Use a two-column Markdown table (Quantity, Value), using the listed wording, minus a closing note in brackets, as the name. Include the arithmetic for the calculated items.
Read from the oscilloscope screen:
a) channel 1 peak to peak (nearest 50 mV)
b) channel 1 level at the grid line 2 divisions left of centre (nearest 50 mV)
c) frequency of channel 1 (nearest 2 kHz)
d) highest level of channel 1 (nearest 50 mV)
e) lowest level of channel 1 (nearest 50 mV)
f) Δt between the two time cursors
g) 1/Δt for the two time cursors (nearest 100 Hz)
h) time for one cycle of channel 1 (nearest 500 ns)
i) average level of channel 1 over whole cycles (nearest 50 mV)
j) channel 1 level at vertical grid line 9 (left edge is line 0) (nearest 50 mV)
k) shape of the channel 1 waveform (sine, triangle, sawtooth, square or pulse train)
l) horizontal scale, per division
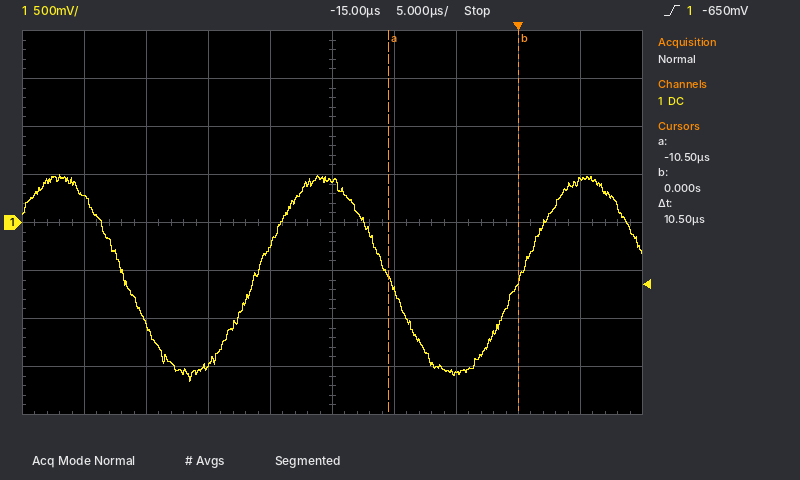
| Quantity | Value |
|---|---|
| channel 1 peak to peak | 500 mV − (-1.65 V) = 2.15 V |
| channel 1 level at the grid line 2 divisions left of centre | -1.50 V |
| frequency of channel 1 | 1 / 21.5 µs ≈ 46 kHz |
| highest level of channel 1 | 500 mV |
| lowest level of channel 1 | -1.65 V |
| Δt between the two time cursors | 10.5 µs |
| 1/Δt for the two time cursors | 1 / 10.5 µs ≈ 95.2 kHz |
| time for one cycle of channel 1 | 21.5 µs |
| average level of channel 1 over whole cycles | (500 mV + (-1.65 V)) / 2 ≈ -575 mV, so -550 mV to the nearest 50 mV |
| channel 1 level at vertical grid line 9 (left edge is line 0) | 450 mV |
| shape of the channel 1 waveform | sine |
| horizontal scale, per division | 5 µs |
